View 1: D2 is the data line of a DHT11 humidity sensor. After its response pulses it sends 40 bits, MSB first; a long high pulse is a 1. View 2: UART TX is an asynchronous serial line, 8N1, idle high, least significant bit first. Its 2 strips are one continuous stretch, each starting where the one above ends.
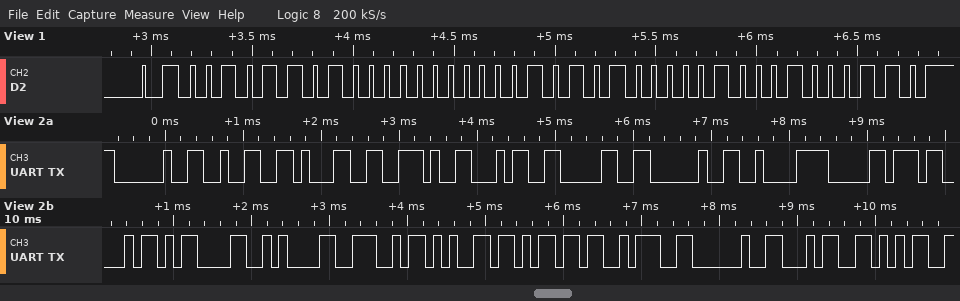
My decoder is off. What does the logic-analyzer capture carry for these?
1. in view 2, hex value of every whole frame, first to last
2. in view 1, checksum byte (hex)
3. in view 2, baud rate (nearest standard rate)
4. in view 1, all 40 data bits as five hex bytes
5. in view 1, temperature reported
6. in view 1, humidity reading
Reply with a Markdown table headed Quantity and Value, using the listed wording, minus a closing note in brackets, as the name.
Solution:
| Quantity | Value |
|---|---|
| in view 2, hex value of every whole frame, first to last | 20 32 31 2E 34 30 20 C2 B0 43 0D 0A 4E 65 6D 3A 20 34 35 |
| in view 1, checksum byte | 0x46 |
| in view 2, baud rate | 9600 baud |
| in view 1, all 40 data bits as five hex bytes | 2D 00 15 04 46 |
| in view 1, temperature reported | 21.4 °C |
| in view 1, humidity reading | 45 % |
